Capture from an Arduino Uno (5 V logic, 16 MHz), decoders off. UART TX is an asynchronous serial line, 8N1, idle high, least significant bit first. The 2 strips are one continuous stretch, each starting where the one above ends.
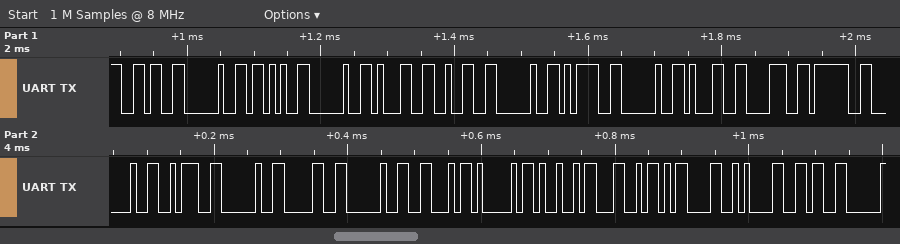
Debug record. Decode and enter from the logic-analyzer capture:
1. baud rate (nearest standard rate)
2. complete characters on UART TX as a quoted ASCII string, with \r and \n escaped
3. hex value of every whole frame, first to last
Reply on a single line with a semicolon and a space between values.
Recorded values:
115200 baud; "6 + 12 = 18? : 0 FAIL\r\n6"; 0x36 0x20 0x2B 0x20 0x31 0x32 0x20 0x3D 0x20 0x31 0x38 0x3F 0x20 0x3A 0x20 0x30 0x20 0x46 0x41 0x49 0x4C 0x0D 0x0A 0x36
